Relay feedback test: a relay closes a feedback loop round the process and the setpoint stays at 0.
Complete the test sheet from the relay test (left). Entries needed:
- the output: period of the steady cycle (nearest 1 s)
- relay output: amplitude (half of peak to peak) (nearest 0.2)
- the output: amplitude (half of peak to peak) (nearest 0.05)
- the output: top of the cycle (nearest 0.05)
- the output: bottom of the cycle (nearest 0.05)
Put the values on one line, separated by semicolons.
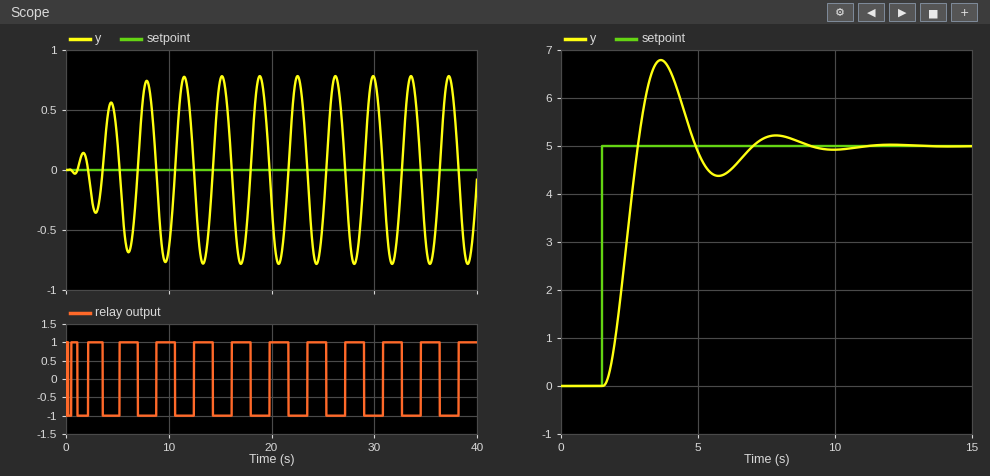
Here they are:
4 s; 1.0; 0.80; 0.80; -0.80
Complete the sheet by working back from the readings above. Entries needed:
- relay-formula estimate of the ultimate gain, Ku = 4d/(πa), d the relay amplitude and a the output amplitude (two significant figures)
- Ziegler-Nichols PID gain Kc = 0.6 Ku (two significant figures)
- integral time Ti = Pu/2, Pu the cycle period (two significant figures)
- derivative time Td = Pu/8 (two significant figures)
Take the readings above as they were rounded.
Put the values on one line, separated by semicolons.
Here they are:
1.6; 0.96; 2.0 s; 0.50 s
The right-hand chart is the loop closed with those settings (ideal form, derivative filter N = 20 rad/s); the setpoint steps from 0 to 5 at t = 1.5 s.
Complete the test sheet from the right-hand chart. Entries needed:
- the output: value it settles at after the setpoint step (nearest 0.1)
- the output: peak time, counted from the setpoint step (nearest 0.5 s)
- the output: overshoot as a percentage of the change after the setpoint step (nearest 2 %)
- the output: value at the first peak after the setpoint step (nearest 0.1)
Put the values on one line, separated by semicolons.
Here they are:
5.0; 2.0 s; 36 %; 6.8
